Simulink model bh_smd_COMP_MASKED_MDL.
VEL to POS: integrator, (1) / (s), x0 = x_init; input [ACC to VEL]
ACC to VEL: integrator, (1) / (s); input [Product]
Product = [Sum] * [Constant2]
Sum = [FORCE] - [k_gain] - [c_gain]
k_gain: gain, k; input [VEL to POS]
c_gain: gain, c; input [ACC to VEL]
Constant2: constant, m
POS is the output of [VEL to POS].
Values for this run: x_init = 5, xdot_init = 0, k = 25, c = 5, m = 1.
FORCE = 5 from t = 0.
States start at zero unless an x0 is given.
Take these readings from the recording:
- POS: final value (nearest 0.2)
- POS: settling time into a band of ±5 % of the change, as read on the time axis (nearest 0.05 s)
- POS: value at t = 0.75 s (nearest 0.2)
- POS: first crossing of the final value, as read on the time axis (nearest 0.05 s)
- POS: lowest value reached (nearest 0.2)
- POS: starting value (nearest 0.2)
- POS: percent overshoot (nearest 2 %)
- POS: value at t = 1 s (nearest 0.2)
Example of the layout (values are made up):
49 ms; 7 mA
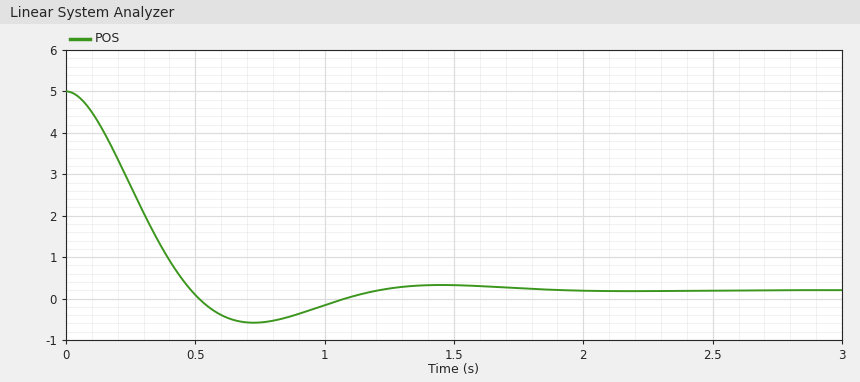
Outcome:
0.2; 1.05 s; -0.6; 0.50 s; -0.6; 5.0; 16 %; -0.2
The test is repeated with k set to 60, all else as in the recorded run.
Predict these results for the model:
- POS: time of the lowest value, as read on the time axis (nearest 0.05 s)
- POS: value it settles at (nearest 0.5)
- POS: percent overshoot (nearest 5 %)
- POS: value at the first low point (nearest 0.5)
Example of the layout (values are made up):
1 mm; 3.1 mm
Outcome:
0.45 s; 0.0; 35 %; -1.5
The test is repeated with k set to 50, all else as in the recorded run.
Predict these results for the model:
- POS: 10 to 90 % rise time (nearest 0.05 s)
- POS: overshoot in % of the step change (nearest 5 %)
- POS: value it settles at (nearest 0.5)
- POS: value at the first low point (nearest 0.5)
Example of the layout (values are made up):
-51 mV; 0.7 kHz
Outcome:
0.20 s; 30 %; 0.0; -1.5
